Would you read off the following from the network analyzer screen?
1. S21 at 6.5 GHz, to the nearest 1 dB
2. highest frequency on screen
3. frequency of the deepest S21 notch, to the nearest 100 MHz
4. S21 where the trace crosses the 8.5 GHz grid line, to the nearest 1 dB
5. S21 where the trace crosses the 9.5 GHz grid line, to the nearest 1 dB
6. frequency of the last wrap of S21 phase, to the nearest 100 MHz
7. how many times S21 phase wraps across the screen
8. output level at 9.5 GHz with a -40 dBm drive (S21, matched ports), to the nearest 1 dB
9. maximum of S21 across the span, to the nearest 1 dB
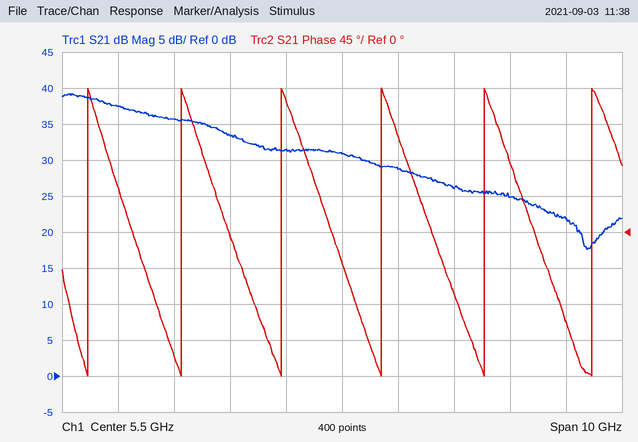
29 dB
10.5 GHz
9.9 GHz
25 dB
22 dB
10.0 GHz
6
-18 dBm
39 dB
